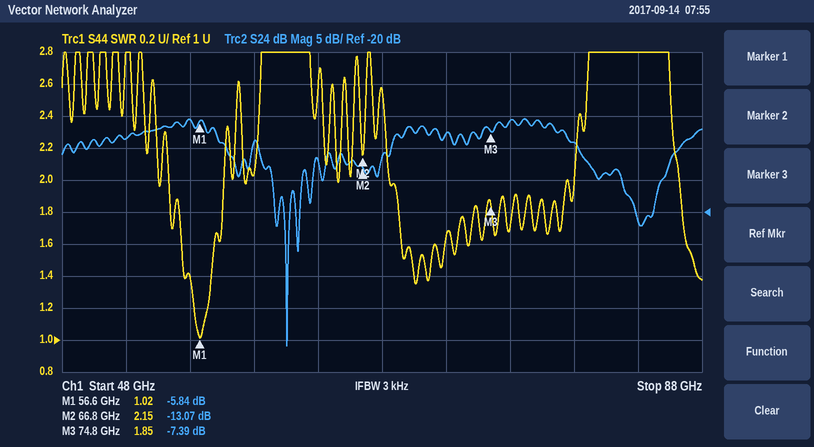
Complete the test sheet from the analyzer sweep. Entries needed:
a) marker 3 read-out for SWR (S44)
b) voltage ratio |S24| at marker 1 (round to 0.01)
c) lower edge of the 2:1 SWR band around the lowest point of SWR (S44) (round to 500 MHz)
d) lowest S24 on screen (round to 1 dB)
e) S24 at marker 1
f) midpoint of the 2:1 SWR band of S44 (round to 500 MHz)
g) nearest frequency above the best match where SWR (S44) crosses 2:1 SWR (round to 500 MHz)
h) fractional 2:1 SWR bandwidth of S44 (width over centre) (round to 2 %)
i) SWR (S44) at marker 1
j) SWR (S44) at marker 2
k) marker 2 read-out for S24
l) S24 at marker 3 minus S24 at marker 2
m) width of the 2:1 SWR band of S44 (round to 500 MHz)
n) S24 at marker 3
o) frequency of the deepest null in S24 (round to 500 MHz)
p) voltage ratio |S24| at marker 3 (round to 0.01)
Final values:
1.85
0.51
54.5 GHz
-41 dB
-5.84 dB
56.5 GHz
58.0 GHz
6 %
1.02
2.15
-13.07 dB
5.68 dB
3.5 GHz
-7.39 dB
62.0 GHz
0.43
